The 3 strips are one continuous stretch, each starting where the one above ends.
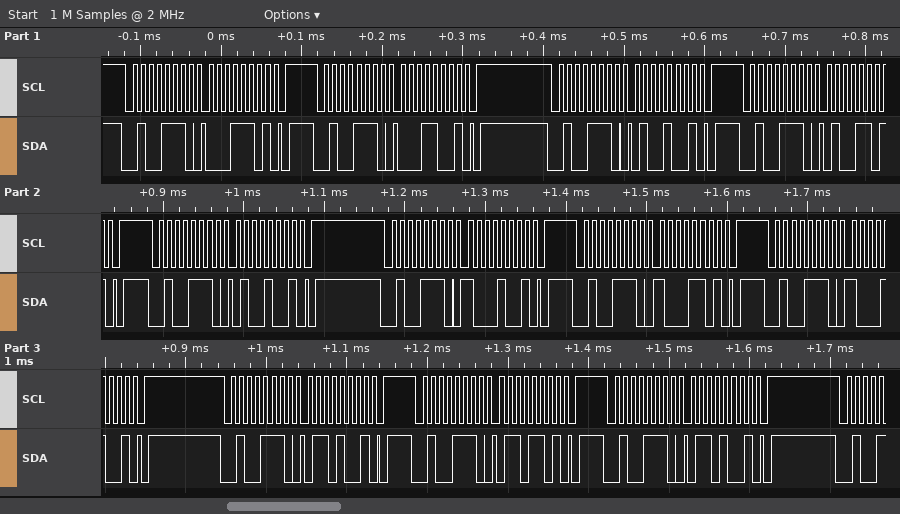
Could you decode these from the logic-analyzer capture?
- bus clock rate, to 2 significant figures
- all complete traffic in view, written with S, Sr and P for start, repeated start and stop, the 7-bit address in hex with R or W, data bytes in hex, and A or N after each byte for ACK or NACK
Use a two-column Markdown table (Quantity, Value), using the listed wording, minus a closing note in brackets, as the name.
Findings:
| Quantity | Value |
|---|---|
| bus clock rate, to 2 significant figures | 100 kHz |
| all complete traffic in view, written with S, Sr and P for start, repeated start and stop, the 7-bit address in hex with R or W, data bytes in hex, and A or N after each byte for ACK or NACK | S 27W A 1D A P S 27W A 19 A P S 27W A 49 A P S 27W A 4D A P S 27W A 49 A P S 27W A 89 A P S 27W A 8D A P S 27W A 89 A P S 27W A 69 A P S 27W A 6D A P S 27W A 69 A P |
